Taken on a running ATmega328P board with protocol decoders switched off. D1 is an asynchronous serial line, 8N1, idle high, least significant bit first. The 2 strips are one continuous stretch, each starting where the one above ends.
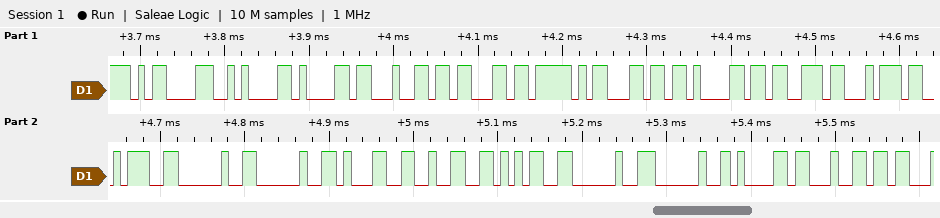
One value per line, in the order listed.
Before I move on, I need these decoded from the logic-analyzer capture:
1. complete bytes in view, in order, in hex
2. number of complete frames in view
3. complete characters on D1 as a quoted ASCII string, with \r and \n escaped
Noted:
0D 0A 61 64 63 5F 6C 61 73 74 3A 20 20 31 32 35 20 20 61 64
20
"\r\nadc_last:  125  ad"
